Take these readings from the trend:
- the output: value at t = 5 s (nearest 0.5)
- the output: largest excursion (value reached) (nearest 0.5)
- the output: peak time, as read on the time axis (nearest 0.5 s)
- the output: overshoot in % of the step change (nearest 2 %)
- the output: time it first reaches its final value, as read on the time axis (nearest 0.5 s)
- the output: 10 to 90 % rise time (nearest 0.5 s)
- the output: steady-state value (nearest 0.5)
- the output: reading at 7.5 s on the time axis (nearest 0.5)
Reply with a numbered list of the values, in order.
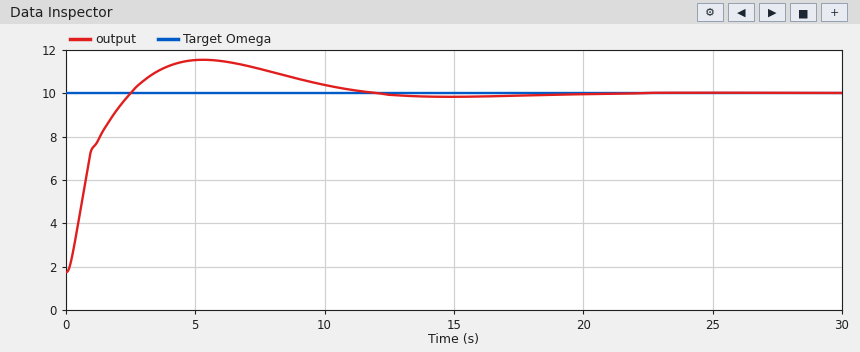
1. 11.5
2. 11.5
3. 5.5 s
4. 18 %
5. 2.5 s
6. 1.5 s
7. 10.0
8. 11.0
